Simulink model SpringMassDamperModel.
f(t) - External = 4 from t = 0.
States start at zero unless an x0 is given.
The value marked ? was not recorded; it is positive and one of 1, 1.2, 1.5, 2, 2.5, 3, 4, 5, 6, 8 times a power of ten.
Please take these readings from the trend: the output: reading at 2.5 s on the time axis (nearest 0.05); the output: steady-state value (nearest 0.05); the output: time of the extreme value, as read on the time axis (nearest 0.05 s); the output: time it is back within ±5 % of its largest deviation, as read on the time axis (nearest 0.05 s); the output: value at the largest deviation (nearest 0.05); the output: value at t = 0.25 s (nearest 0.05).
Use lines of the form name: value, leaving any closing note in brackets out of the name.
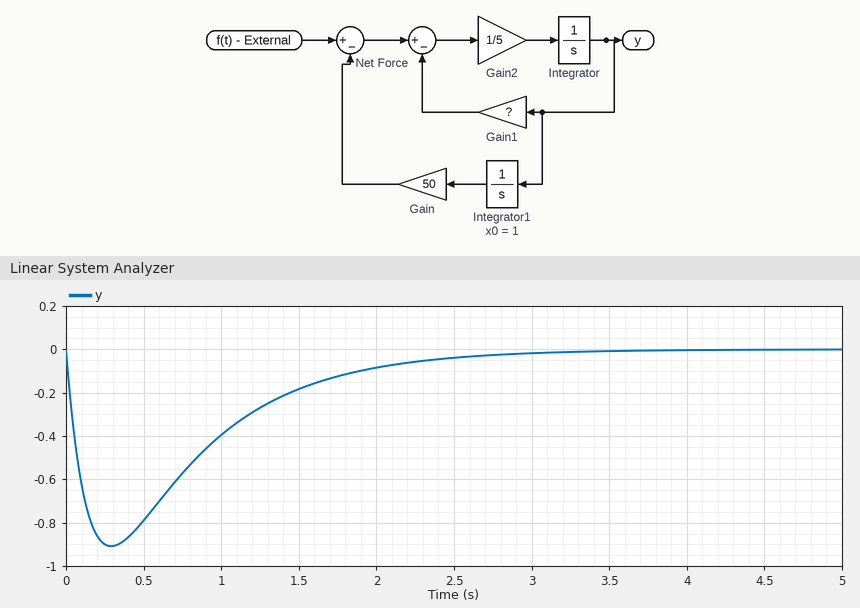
the output: reading at 2.5 s on the time axis: -0.05
the output: steady-state value: 0.00
the output: time of the extreme value, as read on the time axis: 0.30 s
the output: time it is back within ±5 % of its largest deviation, as read on the time axis: 2.40 s
the output: value at the largest deviation: -0.90
the output: value at t = 0.25 s: -0.90
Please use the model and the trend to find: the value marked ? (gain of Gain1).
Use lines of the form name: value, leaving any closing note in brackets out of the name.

the value marked ?: 40
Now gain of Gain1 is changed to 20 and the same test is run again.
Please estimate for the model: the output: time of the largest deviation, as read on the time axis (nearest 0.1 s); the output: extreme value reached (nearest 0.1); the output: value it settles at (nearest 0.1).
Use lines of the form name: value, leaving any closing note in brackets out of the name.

the output: time of the largest deviation, as read on the time axis: 0.4 s
the output: extreme value reached: -1.4
the output: value it settles at: 0.0
